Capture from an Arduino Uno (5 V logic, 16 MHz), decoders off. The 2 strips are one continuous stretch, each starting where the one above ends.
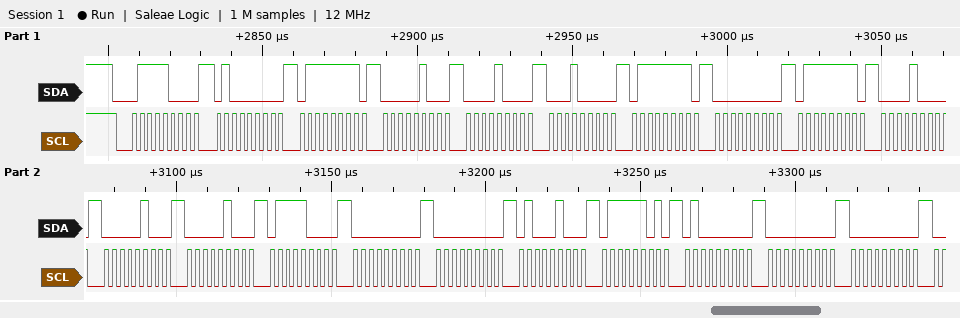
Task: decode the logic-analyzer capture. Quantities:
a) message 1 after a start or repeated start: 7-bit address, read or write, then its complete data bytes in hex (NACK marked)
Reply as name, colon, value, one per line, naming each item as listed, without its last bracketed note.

message 1 after a start or repeated start: 7-bit address, read or write, then its complete data bytes in hex: 0x3C write: 40 7F 04 08 10 7F 00 7F 08 04 04 78 00 00 44 7D 40 00 00
